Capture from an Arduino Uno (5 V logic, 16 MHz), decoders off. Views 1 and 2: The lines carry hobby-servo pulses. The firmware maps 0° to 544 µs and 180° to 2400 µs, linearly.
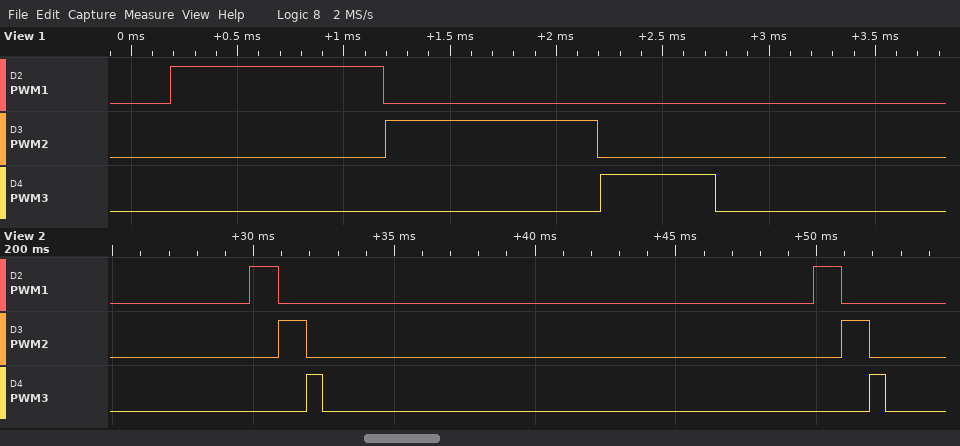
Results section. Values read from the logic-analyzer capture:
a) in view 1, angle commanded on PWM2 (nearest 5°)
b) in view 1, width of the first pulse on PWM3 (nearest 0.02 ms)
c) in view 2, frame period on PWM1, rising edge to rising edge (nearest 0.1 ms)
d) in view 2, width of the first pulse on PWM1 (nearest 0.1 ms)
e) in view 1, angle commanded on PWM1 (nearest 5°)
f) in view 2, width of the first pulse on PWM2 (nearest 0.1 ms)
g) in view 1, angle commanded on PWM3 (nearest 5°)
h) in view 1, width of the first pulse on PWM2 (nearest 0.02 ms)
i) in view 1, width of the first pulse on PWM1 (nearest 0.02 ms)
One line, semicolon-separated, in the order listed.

45°; 0.54 ms; 20.0 ms; 1.0 ms; 45°; 1.0 ms; 0°; 1.00 ms; 1.00 ms
